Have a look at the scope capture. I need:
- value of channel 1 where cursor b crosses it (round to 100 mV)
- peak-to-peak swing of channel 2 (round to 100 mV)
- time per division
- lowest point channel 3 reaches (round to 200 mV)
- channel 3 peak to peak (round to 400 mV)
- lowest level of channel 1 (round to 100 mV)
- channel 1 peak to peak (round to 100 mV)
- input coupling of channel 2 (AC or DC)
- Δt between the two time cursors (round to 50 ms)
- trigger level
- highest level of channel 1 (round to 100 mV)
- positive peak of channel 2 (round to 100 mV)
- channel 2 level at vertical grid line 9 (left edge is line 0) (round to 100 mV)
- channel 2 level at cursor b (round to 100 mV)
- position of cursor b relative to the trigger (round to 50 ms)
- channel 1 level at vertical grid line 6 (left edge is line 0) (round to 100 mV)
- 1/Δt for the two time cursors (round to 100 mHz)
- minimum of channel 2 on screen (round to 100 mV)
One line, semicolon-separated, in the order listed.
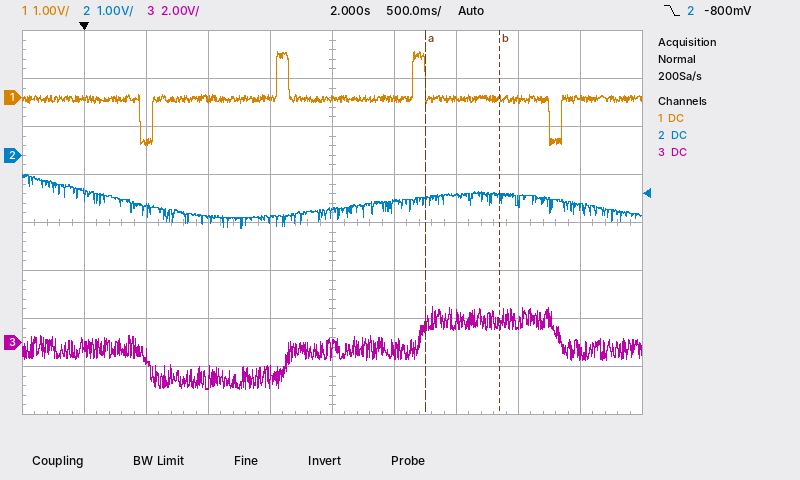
0.0 V; 1.1 V; 500 ms; -2.0 V; 3.6 V; -1.0 V; 2.0 V; DC; 600 ms; -800 mV; 1.0 V; -400 mV; -1.1 V; -900 mV; +3.35 s; 0.0 V; 1.7 Hz; -1.5 V
